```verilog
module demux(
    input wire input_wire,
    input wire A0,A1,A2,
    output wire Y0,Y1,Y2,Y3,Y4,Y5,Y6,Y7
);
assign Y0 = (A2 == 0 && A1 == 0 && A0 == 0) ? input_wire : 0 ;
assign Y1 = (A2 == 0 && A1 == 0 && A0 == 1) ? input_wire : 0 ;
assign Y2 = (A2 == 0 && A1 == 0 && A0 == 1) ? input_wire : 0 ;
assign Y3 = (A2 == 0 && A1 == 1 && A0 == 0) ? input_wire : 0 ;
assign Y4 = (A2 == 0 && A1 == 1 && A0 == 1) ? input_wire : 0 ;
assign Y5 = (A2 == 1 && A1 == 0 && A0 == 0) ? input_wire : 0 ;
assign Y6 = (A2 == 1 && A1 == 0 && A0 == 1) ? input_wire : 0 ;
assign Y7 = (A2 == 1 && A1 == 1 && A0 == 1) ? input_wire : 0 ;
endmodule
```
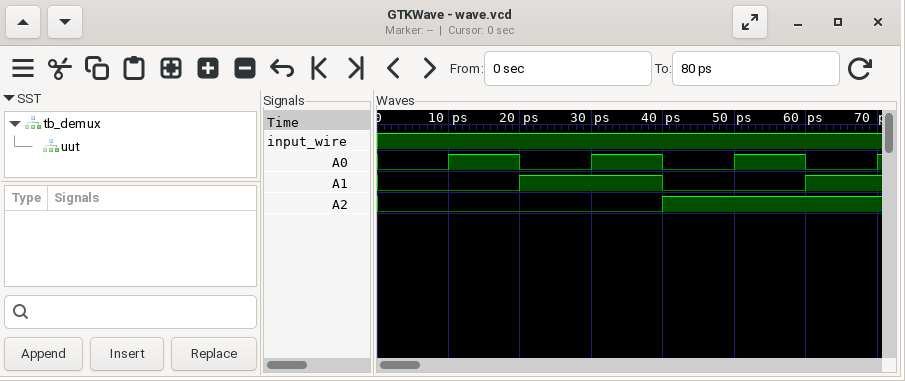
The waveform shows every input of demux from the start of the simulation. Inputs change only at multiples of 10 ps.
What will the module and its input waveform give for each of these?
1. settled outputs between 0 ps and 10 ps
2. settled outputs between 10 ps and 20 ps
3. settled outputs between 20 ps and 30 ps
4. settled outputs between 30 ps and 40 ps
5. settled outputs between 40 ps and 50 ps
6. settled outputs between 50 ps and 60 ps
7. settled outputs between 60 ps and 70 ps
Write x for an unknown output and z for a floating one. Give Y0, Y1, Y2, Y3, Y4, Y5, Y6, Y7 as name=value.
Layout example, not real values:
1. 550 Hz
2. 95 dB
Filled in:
1. Y0=1, Y1=0, Y2=0, Y3=0, Y4=0, Y5=0, Y6=0, Y7=0
2. Y0=0, Y1=1, Y2=1, Y3=0, Y4=0, Y5=0, Y6=0, Y7=0
3. Y0=0, Y1=0, Y2=0, Y3=1, Y4=0, Y5=0, Y6=0, Y7=0
4. Y0=0, Y1=0, Y2=0, Y3=0, Y4=1, Y5=0, Y6=0, Y7=0
5. Y0=0, Y1=0, Y2=0, Y3=0, Y4=0, Y5=1, Y6=0, Y7=0
6. Y0=0, Y1=0, Y2=0, Y3=0, Y4=0, Y5=0, Y6=1, Y7=0
7. Y0=0, Y1=0, Y2=0, Y3=0, Y4=0, Y5=0, Y6=0, Y7=0
